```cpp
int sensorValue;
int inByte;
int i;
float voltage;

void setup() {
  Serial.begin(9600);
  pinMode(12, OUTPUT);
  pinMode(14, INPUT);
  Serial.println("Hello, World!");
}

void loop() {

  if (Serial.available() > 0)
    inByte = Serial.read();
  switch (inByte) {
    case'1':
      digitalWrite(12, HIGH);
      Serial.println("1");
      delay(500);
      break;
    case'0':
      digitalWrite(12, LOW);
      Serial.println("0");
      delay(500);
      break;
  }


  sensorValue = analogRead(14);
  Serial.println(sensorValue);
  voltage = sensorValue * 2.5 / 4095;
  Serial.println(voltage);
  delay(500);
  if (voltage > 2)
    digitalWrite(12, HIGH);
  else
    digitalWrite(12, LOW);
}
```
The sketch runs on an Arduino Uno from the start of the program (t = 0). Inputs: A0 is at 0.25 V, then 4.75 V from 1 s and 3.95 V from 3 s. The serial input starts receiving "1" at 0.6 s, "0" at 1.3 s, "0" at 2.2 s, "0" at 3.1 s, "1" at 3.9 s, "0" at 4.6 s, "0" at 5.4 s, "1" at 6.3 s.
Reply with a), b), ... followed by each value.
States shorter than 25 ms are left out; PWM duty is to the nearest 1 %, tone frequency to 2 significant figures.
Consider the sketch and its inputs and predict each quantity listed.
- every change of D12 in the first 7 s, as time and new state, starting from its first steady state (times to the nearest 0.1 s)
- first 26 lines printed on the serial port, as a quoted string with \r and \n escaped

a) 0 s low; 1 s high; 2 s low; 5 s high; 6 s low
b) "Hello, World!\r\n51\r\n0.03\r\n51\r\n0.03\r\n1\r\n972\r\n0.59\r\n0\r\n972\r\n0.59\r\n0\r\n808\r\n0.49\r\n0\r\n808\r\n0.49\r\n1\r\n808\r\n0.49\r\n0\r\n808\r\n0.49\r\n0\r\n808\r\n0.49\r\n"
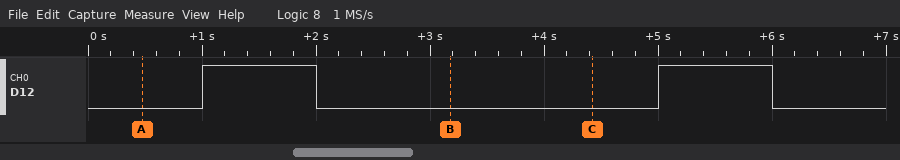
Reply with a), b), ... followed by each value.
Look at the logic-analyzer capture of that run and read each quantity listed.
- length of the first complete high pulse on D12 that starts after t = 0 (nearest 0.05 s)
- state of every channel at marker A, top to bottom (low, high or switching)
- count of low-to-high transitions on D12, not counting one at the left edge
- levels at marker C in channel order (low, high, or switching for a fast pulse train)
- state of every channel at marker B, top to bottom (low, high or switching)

a) 1.00 s
b) D12 low
c) 2
d) D12 low
e) D12 low
